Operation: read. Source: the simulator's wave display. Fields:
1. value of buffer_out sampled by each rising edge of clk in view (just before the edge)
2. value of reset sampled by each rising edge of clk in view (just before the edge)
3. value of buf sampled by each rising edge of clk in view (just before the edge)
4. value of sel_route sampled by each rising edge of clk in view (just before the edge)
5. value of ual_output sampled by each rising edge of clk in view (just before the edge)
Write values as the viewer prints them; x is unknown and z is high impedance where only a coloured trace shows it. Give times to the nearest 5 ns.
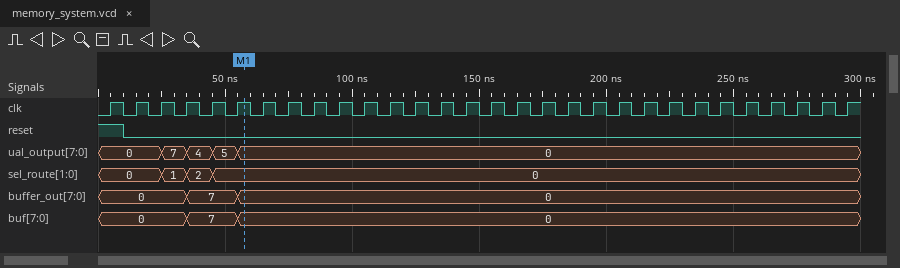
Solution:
0, 0, 0, 0, 7, 7, 0, 0, 0, 0, 0, 0, 0, 0, 0, 0, 0, 0, 0, 0, 0, 0, 0, 0, 0, 0, 0, 0, 0, 0
1 0 0 0 0 0 0 0 0 0 0 0 0 0 0 0 0 0 0 0 0 0 0 0 0 0 0 0 0 0
0, 0, 0, 0, 7, 7, 0, 0, 0, 0, 0, 0, 0, 0, 0, 0, 0, 0, 0, 0, 0, 0, 0, 0, 0, 0, 0, 0, 0, 0
0, 0, 0, 1, 2, 0, 0, 0, 0, 0, 0, 0, 0, 0, 0, 0, 0, 0, 0, 0, 0, 0, 0, 0, 0, 0, 0, 0, 0, 0
0, 0, 0, 7, 4, 5, 0, 0, 0, 0, 0, 0, 0, 0, 0, 0, 0, 0, 0, 0, 0, 0, 0, 0, 0, 0, 0, 0, 0, 0
